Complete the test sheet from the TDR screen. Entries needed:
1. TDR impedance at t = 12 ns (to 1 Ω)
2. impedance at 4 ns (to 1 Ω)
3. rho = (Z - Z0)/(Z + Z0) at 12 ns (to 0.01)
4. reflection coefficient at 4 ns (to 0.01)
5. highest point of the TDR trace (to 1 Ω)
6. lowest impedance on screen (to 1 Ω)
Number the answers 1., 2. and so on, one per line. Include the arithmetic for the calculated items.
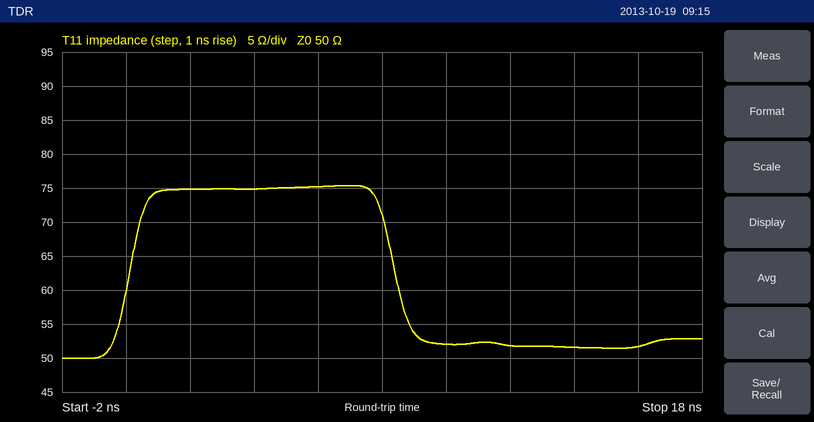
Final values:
1. 52 Ω
2. 75 Ω
3. (52 − 50)/(52 + 50) ≈ +0.02
4. (75 − 50)/(75 + 50) ≈ +0.20
5. 75 Ω
6. 50 Ω
